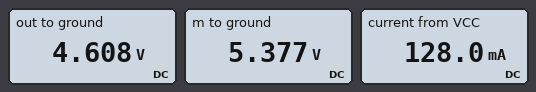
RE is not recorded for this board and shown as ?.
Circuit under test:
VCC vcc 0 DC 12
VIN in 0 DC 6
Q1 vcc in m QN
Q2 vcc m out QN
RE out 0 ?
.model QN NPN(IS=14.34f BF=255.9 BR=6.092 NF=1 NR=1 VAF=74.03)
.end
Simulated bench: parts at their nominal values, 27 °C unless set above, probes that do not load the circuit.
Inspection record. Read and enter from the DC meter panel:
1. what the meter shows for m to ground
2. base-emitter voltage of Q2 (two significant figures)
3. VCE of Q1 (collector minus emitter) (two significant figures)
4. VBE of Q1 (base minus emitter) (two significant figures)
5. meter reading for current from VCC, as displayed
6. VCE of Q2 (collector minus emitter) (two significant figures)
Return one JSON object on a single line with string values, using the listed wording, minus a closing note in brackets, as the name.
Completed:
{"what the meter shows for m to ground": "5.377 V", "base-emitter voltage of Q2": "770 mV", "VCE of Q1 (collector minus emitter)": "6.6 V", "VBE of Q1 (base minus emitter)": "620 mV", "meter reading for current from VCC, as displayed": "128.0 mA", "VCE of Q2 (collector minus emitter)": "7.4 V"}
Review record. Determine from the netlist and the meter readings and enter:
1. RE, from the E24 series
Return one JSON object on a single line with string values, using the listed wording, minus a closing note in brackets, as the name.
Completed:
{"RE, from the E24 series": "36 Ω"}
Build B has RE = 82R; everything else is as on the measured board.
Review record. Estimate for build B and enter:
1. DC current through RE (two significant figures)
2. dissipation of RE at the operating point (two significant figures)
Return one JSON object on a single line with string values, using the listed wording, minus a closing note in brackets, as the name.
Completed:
{"DC current through RE": "57 mA", "dissipation of RE at the operating point": "260 mW"}
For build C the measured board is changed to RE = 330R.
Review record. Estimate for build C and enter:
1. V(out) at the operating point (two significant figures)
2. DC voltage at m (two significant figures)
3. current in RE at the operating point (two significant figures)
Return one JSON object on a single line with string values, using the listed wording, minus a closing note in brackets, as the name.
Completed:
{"V(out) at the operating point": "4.7 V", "DC voltage at m": "5.4 V", "current in RE at the operating point": "14 mA"}
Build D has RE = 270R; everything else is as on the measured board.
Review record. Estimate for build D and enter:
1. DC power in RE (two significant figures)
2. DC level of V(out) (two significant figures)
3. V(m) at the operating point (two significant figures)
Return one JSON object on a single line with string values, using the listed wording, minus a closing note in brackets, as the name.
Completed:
{"DC power in RE": "82 mW", "DC level of V(out)": "4.7 V", "V(m) at the operating point": "5.4 V"}
